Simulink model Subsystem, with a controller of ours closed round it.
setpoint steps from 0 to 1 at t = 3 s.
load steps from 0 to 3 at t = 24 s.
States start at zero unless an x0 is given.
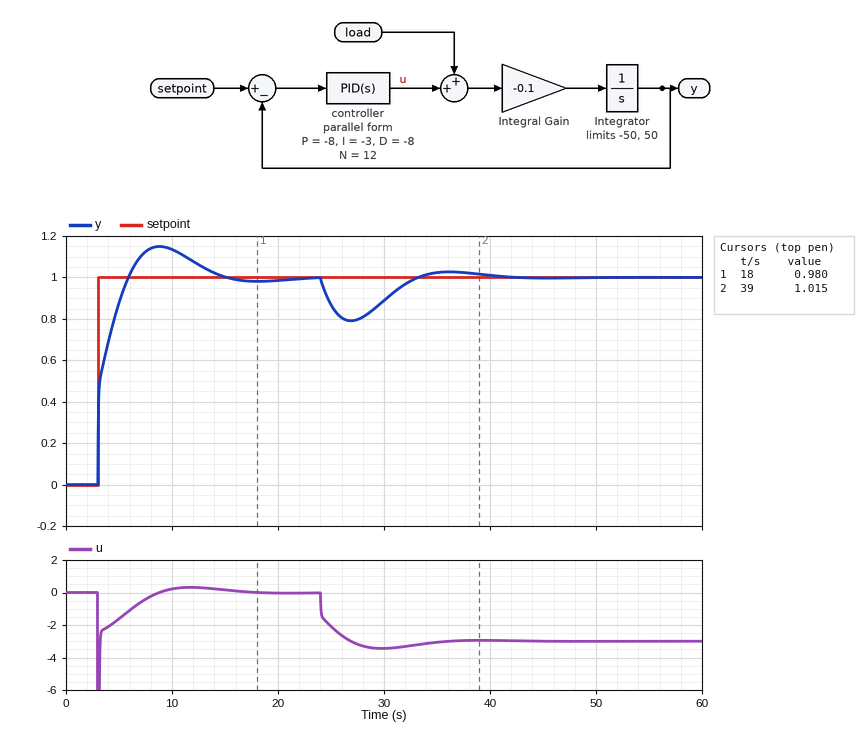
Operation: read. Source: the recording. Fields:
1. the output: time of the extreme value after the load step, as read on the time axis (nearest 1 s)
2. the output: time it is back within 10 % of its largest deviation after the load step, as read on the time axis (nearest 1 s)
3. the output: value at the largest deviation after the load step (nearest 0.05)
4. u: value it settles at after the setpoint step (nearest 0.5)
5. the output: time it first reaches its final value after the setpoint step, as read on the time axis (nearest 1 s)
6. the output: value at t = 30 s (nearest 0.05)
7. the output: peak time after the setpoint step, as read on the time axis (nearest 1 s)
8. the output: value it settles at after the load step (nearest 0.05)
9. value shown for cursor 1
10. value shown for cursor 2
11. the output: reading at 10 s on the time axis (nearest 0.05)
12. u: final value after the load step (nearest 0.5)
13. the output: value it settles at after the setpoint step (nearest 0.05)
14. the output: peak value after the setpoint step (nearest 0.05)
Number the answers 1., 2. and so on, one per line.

1. 27 s
2. 38 s
3. 0.80
4. 0.0
5. 6 s
6. 0.90
7. 9 s
8. 1.00
9. 0.980
10. 1.015
11. 1.15
12. -3.0
13. 1.00
14. 1.15
